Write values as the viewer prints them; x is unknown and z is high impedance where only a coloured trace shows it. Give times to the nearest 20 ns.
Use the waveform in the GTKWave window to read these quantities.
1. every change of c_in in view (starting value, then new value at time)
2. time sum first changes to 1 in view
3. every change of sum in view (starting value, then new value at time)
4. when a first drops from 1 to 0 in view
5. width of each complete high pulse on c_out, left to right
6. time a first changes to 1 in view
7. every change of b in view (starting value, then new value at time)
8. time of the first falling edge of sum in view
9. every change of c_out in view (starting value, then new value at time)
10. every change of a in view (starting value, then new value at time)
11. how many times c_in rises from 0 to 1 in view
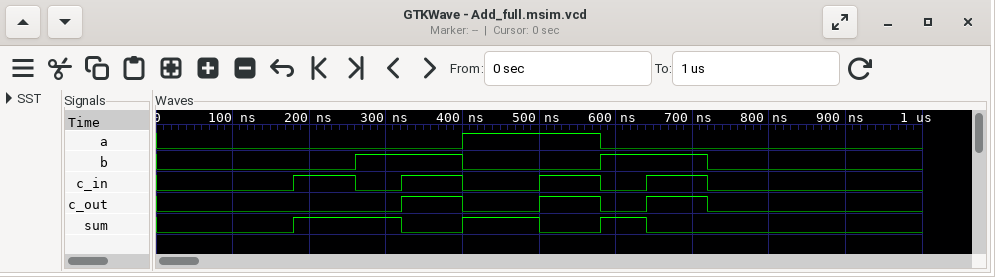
0, 1 at 180 ns, 0 at 260 ns, 1 at 320 ns, 0 at 400 ns, 1 at 500 ns, 0 at 580 ns, 1 at 640 ns, 0 at 720 ns
180 ns
0, 1 at 180 ns, 0 at 320 ns, 1 at 400 ns, 0 at 500 ns, 1 at 580 ns, 0 at 640 ns
580 ns
80 ns, 80 ns, 80 ns
400 ns
0, 1 at 260 ns, 0 at 400 ns, 1 at 580 ns, 0 at 720 ns
320 ns
0, 1 at 320 ns, 0 at 400 ns, 1 at 500 ns, 0 at 580 ns, 1 at 640 ns, 0 at 720 ns
0, 1 at 400 ns, 0 at 580 ns
4
